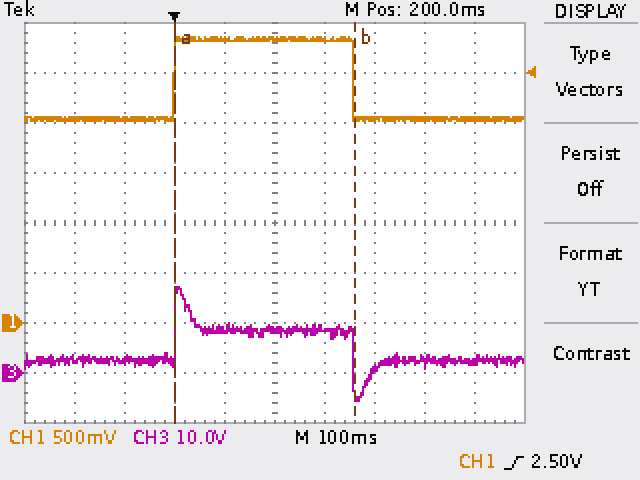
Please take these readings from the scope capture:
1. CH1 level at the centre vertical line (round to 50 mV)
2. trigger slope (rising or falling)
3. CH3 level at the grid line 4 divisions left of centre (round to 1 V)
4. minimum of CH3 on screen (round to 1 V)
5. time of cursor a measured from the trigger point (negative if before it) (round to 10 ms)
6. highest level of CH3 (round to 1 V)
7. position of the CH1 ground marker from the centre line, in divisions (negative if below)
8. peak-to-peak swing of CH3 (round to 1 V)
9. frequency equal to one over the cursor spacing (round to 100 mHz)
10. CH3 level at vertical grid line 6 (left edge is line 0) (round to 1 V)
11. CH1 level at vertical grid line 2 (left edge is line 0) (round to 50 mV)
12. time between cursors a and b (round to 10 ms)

2.85 V
rising
3 V
-6 V
0 ms
17 V
-2.0 div
23 V
2.8 Hz
9 V
2.05 V
360 ms
